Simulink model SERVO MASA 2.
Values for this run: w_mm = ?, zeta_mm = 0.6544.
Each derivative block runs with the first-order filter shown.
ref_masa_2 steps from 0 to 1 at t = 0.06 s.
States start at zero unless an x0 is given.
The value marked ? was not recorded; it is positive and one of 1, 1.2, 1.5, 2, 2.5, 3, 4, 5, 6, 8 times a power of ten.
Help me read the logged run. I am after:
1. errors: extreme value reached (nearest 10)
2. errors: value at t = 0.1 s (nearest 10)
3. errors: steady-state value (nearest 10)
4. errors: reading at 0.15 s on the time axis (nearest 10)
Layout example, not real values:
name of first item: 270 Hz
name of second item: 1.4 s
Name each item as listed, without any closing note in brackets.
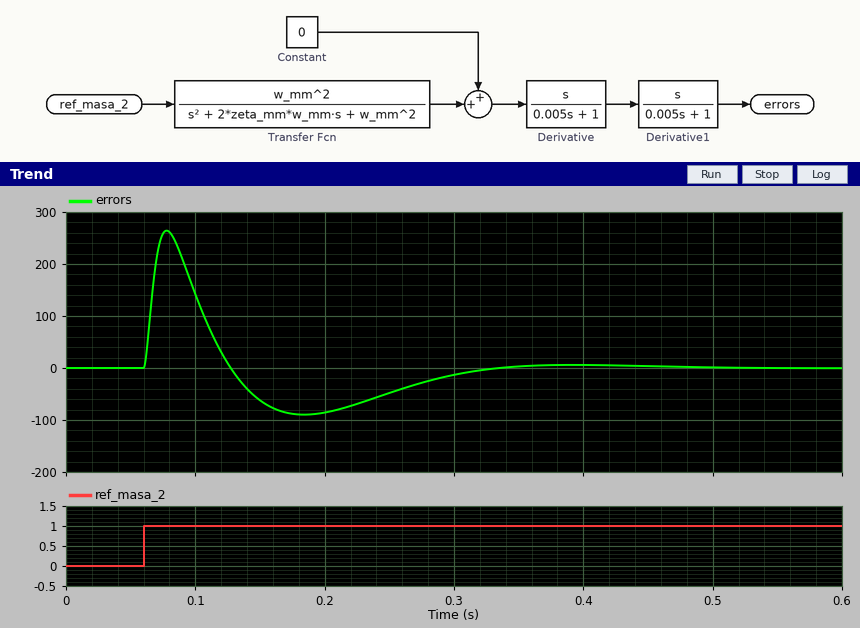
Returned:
errors: extreme value reached: 260
errors: value at t = 0.1 s: 140
errors: steady-state value: 0
errors: reading at 0.15 s on the time axis: -60
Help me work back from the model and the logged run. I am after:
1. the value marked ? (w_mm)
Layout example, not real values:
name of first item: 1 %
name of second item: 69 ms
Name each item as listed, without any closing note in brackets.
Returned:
the value marked ?: 20
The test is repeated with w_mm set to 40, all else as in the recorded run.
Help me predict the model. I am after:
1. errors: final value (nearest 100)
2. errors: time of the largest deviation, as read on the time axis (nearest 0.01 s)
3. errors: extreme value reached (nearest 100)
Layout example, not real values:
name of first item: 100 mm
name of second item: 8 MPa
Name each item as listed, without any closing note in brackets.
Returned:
errors: final value: 0
errors: time of the largest deviation, as read on the time axis: 0.07 s
errors: extreme value reached: 800
